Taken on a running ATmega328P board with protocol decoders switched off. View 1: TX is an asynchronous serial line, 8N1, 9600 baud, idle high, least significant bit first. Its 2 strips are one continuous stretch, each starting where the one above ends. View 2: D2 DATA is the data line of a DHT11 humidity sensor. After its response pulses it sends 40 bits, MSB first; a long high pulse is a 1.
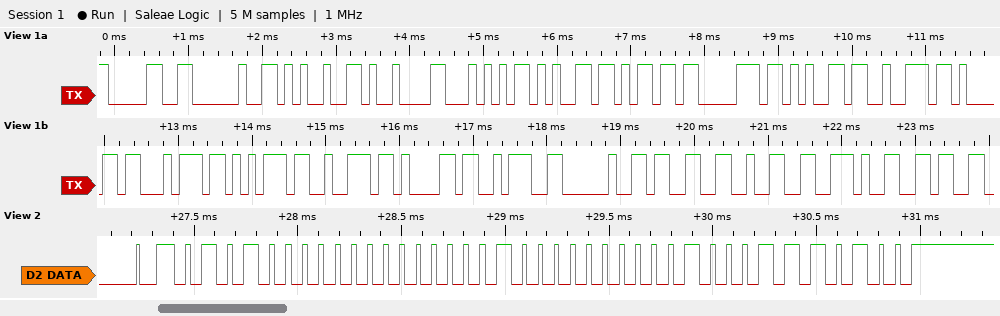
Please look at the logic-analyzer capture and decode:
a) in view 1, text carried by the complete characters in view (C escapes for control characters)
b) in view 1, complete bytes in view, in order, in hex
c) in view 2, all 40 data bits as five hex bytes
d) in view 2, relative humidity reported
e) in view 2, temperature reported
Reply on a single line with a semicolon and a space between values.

"0 %\tTemperatura: 32.6"; 30 20 25 09 54 65 6D 70 65 72 61 74 75 72 61 3A 20 33 32 2E 36; 50 00 20 04 74; 80 %; 32.4 °C
